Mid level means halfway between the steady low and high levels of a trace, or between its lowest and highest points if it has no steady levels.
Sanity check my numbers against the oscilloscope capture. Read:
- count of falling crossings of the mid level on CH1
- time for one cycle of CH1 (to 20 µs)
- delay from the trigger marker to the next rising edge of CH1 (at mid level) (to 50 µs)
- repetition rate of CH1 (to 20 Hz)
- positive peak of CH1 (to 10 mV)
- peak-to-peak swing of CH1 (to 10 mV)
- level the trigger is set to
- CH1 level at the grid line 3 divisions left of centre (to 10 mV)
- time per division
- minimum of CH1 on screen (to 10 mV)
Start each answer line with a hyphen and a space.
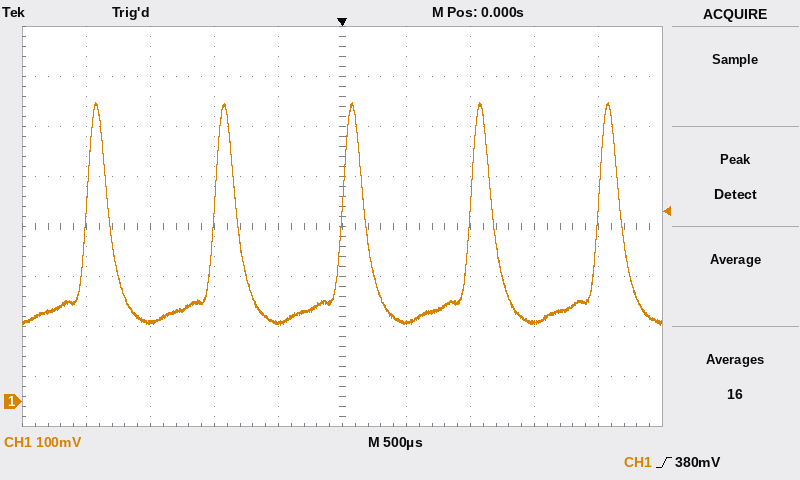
- 5
- 1.00 ms
- 1.00 ms
- 1.00 kHz
- 600 mV
- 450 mV
- 380 mV
- 160 mV
- 500 µs
- 150 mV
